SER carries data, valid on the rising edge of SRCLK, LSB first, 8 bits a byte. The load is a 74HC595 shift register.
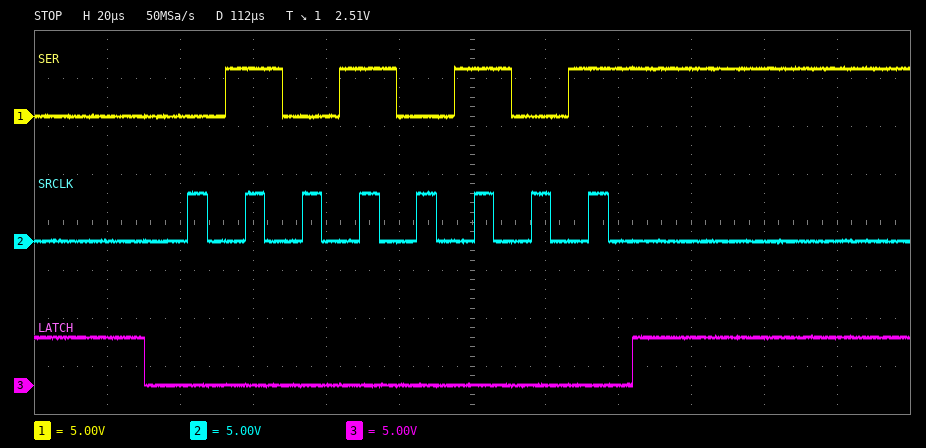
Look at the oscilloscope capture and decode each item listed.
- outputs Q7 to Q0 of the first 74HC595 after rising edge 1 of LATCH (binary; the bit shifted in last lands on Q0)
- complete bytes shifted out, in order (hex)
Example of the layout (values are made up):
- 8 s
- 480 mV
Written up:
- 01010101
- 0xAA
